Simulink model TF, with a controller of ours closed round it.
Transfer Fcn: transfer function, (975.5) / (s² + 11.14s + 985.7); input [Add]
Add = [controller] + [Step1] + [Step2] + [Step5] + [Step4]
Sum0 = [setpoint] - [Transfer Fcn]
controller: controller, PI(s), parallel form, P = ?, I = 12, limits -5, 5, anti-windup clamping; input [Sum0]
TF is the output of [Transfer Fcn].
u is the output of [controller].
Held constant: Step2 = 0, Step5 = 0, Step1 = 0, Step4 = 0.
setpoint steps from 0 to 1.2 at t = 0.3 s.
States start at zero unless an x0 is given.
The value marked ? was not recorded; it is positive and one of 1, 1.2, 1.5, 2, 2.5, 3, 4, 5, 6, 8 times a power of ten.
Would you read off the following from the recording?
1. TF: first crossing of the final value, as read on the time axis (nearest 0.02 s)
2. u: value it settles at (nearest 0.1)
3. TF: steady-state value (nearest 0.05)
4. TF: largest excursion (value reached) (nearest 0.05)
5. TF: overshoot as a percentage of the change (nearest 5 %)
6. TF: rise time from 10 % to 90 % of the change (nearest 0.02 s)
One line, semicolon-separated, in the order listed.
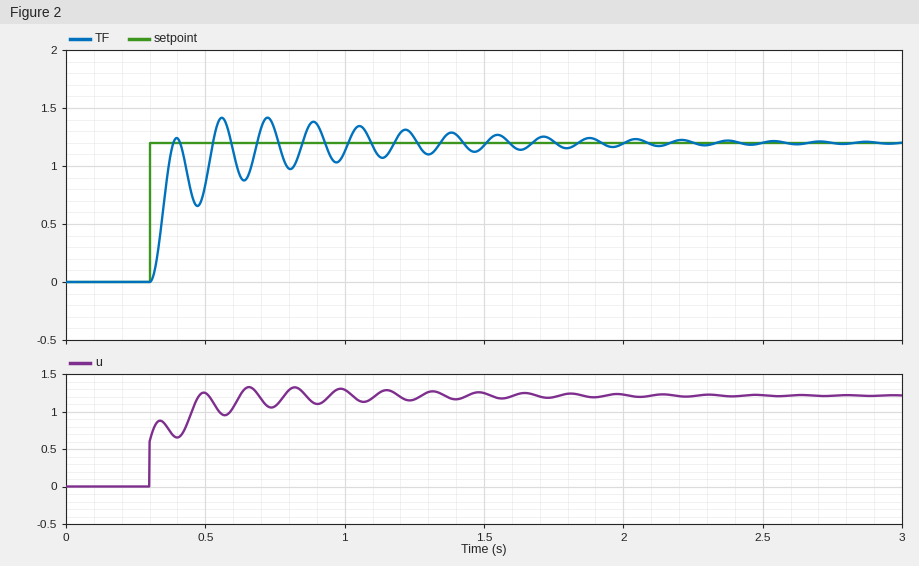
0.38 s; 1.2; 1.20; 1.40; 20 %; 0.06 s
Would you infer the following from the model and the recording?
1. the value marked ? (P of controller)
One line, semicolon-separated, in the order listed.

0.5
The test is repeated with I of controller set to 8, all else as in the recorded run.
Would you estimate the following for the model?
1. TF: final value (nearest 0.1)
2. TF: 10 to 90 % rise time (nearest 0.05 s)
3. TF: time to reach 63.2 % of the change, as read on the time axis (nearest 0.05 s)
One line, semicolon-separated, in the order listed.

1.2; 0.20 s; 0.35 s
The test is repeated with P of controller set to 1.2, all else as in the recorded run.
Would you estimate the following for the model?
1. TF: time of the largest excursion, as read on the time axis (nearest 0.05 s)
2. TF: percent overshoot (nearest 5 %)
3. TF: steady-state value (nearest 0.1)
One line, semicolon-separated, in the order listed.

0.50 s; 15 %; 1.2
